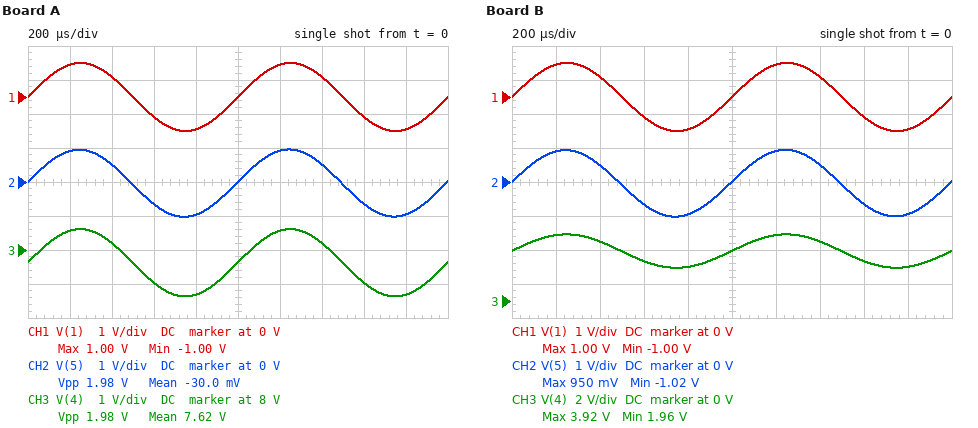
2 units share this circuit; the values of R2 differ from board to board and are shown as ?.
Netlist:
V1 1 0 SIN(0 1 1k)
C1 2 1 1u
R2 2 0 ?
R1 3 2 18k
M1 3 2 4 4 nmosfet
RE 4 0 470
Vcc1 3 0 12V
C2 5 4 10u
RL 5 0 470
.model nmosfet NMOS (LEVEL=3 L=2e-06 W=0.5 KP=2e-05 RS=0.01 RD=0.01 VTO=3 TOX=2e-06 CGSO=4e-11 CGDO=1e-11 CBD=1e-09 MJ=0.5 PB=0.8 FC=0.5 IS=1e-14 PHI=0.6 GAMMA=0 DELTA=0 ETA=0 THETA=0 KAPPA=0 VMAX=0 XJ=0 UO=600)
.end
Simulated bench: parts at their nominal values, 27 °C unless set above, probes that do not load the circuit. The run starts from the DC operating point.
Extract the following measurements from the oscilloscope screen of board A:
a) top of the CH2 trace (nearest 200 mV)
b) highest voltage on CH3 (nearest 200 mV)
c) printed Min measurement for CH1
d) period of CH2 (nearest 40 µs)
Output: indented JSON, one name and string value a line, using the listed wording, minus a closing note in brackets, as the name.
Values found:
{
  "top of the CH2 trace": "1.0 V",
  "highest voltage on CH3": "8.6 V",
  "printed Min measurement for CH1": "-1.00 V",
  "period of CH2": "1.00 ms"
}
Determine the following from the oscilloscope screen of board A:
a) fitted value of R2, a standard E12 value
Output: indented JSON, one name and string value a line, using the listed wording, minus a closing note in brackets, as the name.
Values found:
{
  "fitted value of R2, a standard E12 value": "150 kΩ"
}
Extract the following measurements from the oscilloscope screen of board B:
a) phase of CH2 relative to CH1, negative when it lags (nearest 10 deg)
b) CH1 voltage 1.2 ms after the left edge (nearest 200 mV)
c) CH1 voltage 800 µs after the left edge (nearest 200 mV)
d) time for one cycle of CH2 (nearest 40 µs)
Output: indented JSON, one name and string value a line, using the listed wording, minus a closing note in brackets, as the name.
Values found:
{
  "phase of CH2 relative to CH1, negative when it lags": "0 deg",
  "CH1 voltage 1.2 ms after the left edge": "1.0 V",
  "CH1 voltage 800 µs after the left edge": "-1.0 V",
  "time for one cycle of CH2": "1.00 ms"
}
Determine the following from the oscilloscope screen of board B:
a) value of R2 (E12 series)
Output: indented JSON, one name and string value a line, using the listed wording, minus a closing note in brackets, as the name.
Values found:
{
  "value of R2": "18 kΩ"
}
